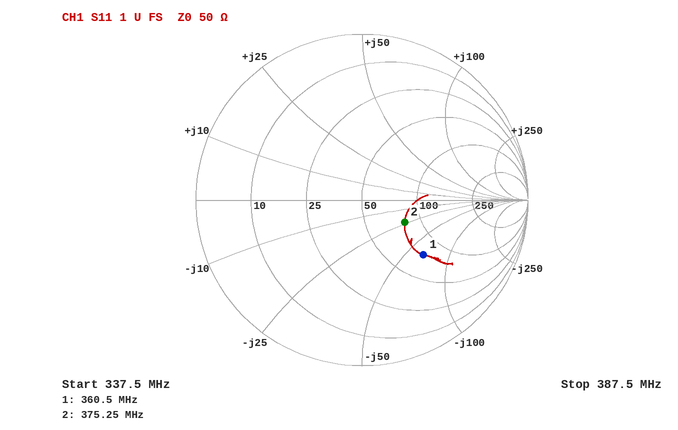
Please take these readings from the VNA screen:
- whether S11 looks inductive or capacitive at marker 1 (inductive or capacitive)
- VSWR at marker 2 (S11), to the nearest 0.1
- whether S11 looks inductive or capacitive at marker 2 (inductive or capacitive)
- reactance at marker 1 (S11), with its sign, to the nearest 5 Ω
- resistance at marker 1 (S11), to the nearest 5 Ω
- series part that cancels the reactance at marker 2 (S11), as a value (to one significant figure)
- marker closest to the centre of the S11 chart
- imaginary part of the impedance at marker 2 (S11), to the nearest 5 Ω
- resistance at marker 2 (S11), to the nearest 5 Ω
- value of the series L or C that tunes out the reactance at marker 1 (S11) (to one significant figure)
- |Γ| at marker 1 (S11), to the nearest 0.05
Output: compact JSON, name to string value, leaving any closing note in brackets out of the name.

{"whether S11 looks inductive or capacitive at marker 1": "capacitive", "VSWR at marker 2 (S11), to the nearest 0.1": "1.8", "whether S11 looks inductive or capacitive at marker 2": "capacitive", "reactance at marker 1 (S11), with its sign, to the nearest 5 Ω": "-65 Ω", "resistance at marker 1 (S11), to the nearest 5 Ω": "75 Ω", "series part that cancels the reactance at marker 2 (S11), as a value": "10 nH", "marker closest to the centre of the S11 chart": "marker 2", "imaginary part of the impedance at marker 2 (S11), to the nearest 5 Ω": "-25 Ω", "resistance at marker 2 (S11), to the nearest 5 Ω": "80 Ω", "value of the series L or C that tunes out the reactance at marker 1 (S11)": "30 nH", "|Γ| at marker 1 (S11), to the nearest 0.05": "0.50"}
